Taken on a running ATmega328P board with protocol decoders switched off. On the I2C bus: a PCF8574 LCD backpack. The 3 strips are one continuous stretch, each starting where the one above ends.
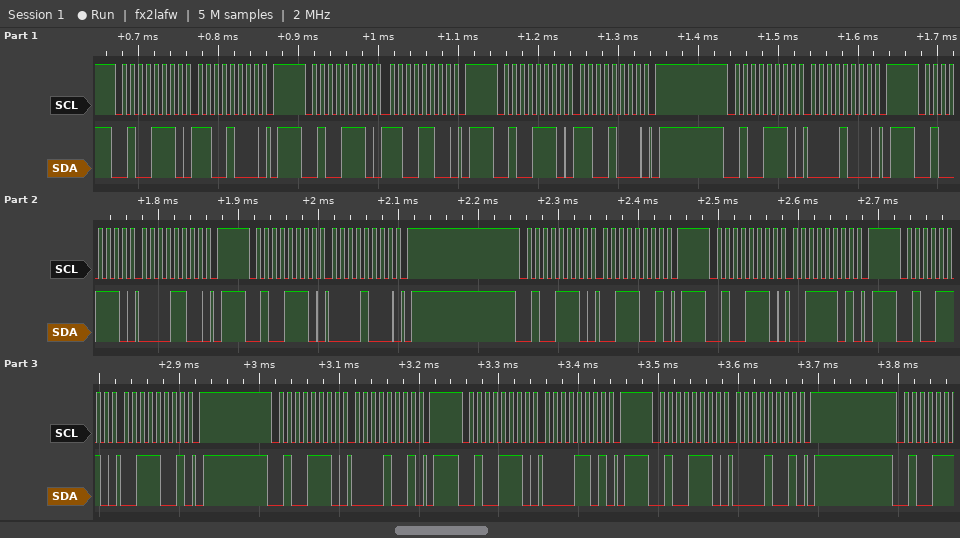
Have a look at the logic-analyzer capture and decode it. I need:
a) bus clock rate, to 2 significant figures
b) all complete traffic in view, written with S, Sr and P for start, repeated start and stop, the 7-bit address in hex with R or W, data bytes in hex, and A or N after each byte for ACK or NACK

100 kHz
S 27W A C8 A P S 27W A CC A P S 27W A C8 A P S 27W A 08 A P S 27W A 0C A P S 27W A 08 A P S 27W A 39 A P S 27W A 3D A P S 27W A 39 A P S 27W A 09 A P S 27W A 0D A P S 27W A 09 A P
